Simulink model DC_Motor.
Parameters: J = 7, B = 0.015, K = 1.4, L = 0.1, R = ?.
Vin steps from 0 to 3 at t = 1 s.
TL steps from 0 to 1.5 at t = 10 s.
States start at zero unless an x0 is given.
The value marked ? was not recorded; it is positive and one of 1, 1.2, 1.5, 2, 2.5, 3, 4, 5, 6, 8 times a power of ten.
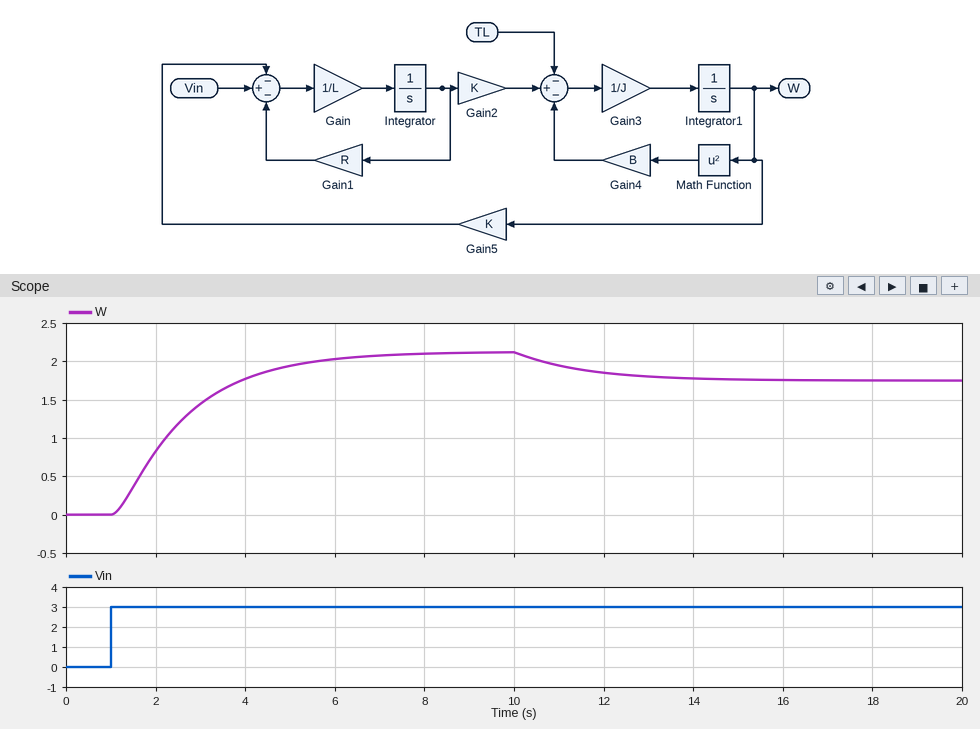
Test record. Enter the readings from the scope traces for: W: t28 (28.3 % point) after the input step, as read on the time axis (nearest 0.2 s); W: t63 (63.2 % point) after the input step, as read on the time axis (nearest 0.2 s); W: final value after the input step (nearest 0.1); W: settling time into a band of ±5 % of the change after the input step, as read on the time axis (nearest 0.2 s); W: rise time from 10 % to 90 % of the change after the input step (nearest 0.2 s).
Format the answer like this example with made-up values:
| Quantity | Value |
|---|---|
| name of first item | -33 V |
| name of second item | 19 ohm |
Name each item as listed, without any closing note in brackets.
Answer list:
| Quantity | Value |
|---|---|
| W: t28 (28.3 % point) after the input step, as read on the time axis | 1.8 s |
| W: t63 (63.2 % point) after the input step, as read on the time axis | 2.8 s |
| W: final value after the input step | 2.1 |
| W: settling time into a band of ±5 % of the change after the input step, as read on the time axis | 5.8 s |
| W: rise time from 10 % to 90 % of the change after the input step | 3.4 s |
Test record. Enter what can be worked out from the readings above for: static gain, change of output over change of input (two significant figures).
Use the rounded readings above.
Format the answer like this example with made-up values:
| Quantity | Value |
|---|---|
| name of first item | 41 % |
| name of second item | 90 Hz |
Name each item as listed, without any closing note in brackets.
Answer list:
| Quantity | Value |
|---|---|
| static gain, change of output over change of input | 0.70 |
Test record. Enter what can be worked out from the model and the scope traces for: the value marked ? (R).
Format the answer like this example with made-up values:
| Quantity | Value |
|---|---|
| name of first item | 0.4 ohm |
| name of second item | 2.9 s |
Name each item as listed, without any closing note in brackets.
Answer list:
| Quantity | Value |
|---|---|
| the value marked ? | 0.5 |
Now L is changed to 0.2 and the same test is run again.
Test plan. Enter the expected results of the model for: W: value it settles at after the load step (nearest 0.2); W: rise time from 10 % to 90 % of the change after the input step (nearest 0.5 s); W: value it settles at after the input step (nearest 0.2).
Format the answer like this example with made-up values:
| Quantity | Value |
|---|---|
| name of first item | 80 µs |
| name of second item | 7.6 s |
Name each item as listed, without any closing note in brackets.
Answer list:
| Quantity | Value |
|---|---|
| W: value it settles at after the load step | 1.8 |
| W: rise time from 10 % to 90 % of the change after the input step | 3.0 s |
| W: value it settles at after the input step | 2.2 |
